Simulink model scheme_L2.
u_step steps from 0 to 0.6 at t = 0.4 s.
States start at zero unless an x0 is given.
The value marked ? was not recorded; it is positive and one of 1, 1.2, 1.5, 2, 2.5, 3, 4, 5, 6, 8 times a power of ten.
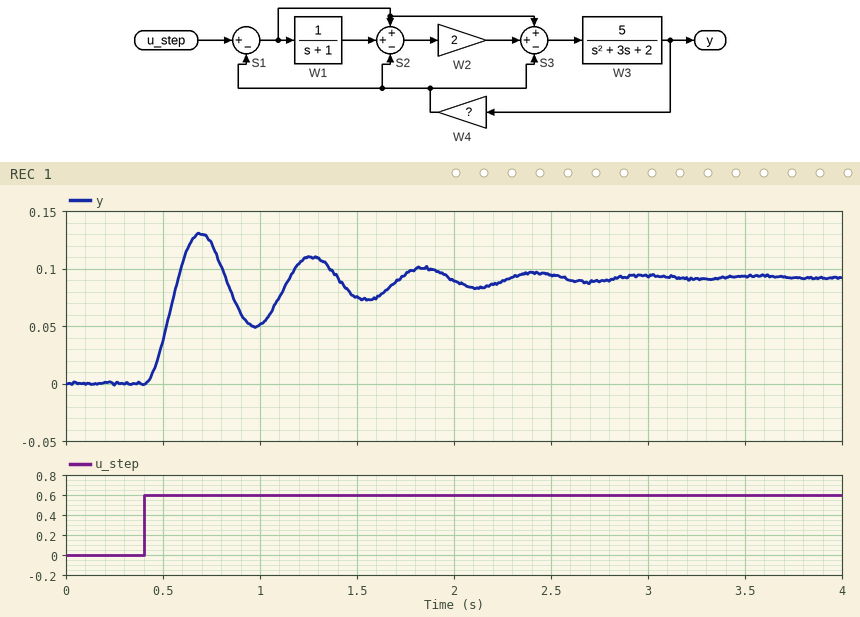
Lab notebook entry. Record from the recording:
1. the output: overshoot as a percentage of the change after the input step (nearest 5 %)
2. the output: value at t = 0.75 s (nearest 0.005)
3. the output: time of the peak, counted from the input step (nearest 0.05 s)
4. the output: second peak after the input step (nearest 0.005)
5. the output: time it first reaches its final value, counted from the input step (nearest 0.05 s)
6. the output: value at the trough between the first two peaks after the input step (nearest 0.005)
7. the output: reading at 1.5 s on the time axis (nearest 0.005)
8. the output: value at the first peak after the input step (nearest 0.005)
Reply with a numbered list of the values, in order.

1. 40 %
2. 0.120
3. 0.30 s
4. 0.110
5. 0.20 s
6. 0.050
7. 0.075
8. 0.130
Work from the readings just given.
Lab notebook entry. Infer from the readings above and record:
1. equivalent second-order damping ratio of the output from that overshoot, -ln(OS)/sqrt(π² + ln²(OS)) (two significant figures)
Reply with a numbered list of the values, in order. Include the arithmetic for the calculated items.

1. ln(0.4) = -0.916; 0.916 / sqrt(9.870 + 0.840) = 0.28
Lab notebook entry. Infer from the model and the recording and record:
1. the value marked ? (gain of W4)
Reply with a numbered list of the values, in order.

1. 4
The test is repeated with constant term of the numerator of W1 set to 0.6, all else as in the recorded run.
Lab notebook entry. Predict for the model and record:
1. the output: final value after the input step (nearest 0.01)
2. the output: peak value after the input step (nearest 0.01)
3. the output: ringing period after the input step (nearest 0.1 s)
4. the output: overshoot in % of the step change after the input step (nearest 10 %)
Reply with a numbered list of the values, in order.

1. 0.09
2. 0.13
3. 0.6 s
4. 50 %
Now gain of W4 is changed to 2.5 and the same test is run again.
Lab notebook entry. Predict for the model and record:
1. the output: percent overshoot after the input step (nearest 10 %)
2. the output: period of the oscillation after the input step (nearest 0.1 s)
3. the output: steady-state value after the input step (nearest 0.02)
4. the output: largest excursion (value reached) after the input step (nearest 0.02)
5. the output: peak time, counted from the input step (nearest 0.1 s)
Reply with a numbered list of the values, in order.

1. 40 %
2. 0.7 s
3. 0.14
4. 0.20
5. 0.4 s
